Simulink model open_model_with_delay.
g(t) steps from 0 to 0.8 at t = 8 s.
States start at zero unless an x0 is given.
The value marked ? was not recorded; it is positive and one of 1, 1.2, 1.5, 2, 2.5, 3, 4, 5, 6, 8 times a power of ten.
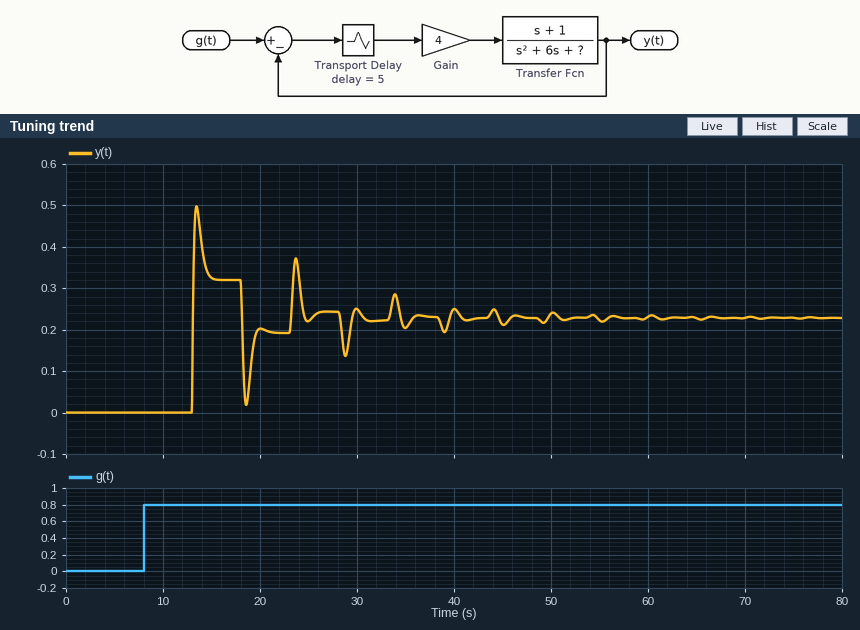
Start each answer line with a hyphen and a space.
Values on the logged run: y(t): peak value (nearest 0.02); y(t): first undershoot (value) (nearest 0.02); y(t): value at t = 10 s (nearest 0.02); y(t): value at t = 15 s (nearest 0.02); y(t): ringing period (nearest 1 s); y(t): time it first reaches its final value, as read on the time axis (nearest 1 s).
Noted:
- 0.50
- 0.02
- 0.00
- 0.32
- 10 s
- 13 s
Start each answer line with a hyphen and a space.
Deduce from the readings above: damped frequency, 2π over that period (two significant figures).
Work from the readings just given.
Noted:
- 0.63 rad/s
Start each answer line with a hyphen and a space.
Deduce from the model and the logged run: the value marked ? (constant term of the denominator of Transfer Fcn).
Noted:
- 10
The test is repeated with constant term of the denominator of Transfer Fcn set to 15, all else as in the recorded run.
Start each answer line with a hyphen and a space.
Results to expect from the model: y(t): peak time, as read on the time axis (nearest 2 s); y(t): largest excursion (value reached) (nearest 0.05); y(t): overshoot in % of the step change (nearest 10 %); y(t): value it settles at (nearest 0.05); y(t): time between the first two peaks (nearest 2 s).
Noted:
- 14 s
- 0.45
- 160 %
- 0.15
- 6 s
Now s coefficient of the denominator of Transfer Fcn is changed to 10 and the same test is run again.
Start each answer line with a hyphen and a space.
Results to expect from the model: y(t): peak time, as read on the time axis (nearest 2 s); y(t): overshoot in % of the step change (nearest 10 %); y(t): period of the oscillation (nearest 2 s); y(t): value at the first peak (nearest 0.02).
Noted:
- 14 s
- 50 %
- 10 s
- 0.34
